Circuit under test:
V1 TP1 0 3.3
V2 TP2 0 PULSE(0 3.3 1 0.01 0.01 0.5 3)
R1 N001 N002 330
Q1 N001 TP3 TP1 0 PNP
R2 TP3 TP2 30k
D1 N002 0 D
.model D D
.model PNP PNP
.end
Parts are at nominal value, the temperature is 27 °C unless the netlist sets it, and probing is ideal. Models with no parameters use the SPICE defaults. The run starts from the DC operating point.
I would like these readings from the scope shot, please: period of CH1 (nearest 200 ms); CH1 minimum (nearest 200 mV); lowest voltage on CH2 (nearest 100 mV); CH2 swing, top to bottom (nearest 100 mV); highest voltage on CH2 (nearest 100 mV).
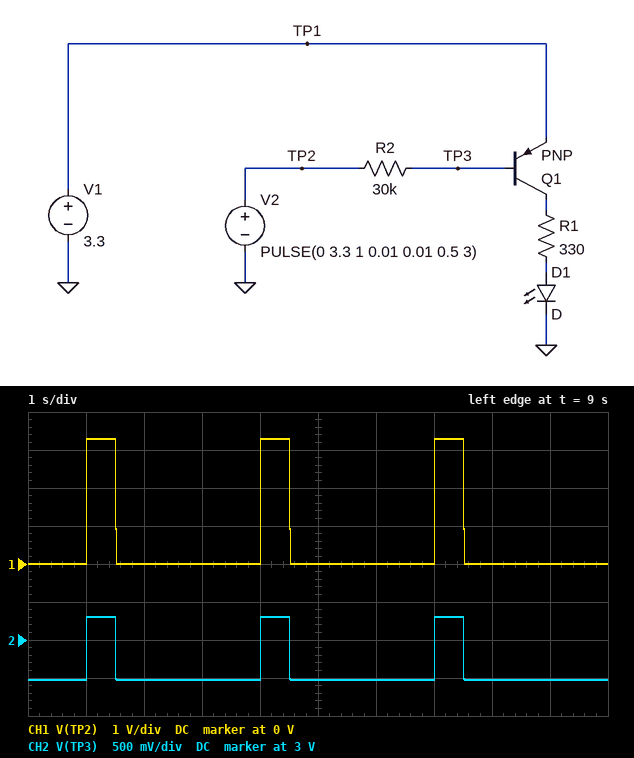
3.0 s
0 V
2.5 V
800 mV
3.3 V
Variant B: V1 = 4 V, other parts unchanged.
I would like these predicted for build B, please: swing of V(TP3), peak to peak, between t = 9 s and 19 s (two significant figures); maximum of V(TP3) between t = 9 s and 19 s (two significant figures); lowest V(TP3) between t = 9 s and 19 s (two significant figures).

140 mV
3.3 V
3.2 V
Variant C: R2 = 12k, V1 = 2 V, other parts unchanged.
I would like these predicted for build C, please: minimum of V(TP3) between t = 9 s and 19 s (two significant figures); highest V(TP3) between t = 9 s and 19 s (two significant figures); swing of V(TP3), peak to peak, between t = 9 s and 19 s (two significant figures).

1.2 V
3.3 V
2.1 V
